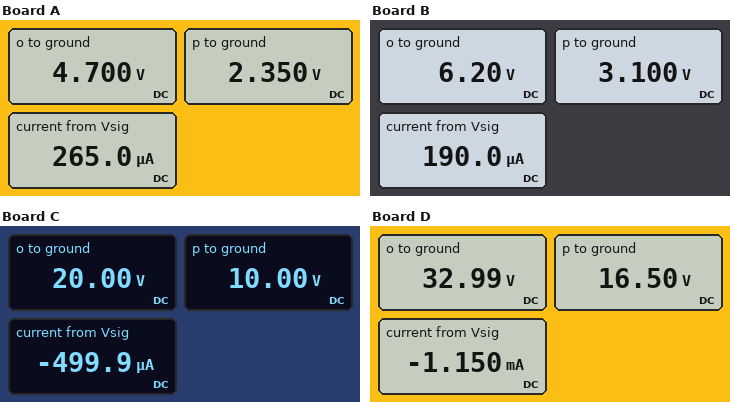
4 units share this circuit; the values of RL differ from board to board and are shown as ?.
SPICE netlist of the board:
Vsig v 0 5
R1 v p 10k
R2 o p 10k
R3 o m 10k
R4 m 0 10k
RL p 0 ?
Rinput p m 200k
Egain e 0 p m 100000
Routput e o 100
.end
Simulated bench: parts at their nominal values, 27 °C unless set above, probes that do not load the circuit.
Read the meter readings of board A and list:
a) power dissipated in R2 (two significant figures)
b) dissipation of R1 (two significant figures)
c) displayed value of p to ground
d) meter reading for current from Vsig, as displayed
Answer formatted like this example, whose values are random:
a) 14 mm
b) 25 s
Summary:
a) 550 µW
b) 700 µW
c) 2.350 V
d) 265.0 µA
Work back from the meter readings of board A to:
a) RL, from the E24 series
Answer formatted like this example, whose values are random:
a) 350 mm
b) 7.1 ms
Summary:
a) 4.7 kΩ
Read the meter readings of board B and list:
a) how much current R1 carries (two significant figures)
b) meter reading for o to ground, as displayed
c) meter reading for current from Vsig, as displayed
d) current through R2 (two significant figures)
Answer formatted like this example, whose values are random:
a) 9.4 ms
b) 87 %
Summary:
a) 190 µA
b) 6.20 V
c) 190.0 µA
d) 310 µA
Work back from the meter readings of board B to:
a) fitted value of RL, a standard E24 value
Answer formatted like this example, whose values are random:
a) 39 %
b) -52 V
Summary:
a) 6.2 kΩ
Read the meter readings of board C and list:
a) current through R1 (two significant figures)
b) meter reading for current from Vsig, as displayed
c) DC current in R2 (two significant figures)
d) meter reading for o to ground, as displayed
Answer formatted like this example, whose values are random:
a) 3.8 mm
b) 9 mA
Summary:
a) 500 µA
b) -499.9 µA
c) 1.0 mA
d) 20.00 V
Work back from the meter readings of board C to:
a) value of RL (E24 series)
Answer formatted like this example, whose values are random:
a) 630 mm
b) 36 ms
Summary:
a) 20 kΩ
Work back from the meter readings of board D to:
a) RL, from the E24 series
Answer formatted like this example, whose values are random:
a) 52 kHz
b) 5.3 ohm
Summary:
a) 33 kΩ
